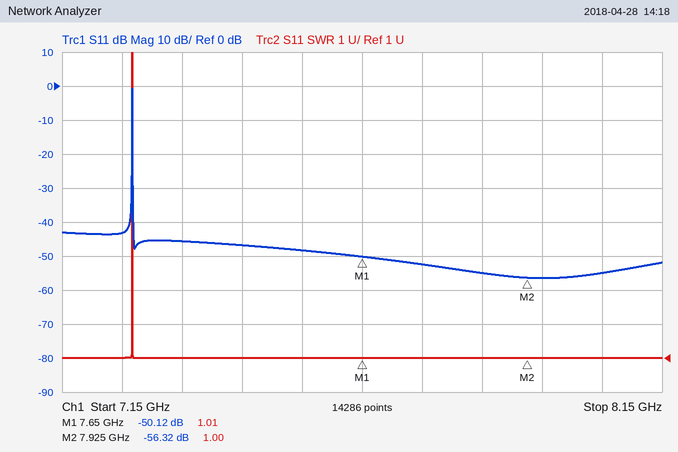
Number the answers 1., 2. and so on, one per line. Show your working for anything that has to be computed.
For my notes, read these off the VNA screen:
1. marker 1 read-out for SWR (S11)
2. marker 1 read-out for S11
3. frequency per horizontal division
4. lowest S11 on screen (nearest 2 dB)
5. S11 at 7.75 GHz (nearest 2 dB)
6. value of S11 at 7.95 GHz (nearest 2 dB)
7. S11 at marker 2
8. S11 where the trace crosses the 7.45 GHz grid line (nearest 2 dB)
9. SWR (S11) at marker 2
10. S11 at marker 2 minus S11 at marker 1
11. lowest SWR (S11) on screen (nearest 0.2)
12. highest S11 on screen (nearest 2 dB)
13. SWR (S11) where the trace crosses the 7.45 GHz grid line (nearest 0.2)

1. 1.01
2. -50.12 dB
3. 100 MHz
4. -56 dB
5. -52 dB
6. -56 dB
7. -56.32 dB
8. -46 dB
9. 1.00
10. -56.32 − (-50.12) = -6.20 dB
11. 1.0
12. 0 dB
13. 1.0
